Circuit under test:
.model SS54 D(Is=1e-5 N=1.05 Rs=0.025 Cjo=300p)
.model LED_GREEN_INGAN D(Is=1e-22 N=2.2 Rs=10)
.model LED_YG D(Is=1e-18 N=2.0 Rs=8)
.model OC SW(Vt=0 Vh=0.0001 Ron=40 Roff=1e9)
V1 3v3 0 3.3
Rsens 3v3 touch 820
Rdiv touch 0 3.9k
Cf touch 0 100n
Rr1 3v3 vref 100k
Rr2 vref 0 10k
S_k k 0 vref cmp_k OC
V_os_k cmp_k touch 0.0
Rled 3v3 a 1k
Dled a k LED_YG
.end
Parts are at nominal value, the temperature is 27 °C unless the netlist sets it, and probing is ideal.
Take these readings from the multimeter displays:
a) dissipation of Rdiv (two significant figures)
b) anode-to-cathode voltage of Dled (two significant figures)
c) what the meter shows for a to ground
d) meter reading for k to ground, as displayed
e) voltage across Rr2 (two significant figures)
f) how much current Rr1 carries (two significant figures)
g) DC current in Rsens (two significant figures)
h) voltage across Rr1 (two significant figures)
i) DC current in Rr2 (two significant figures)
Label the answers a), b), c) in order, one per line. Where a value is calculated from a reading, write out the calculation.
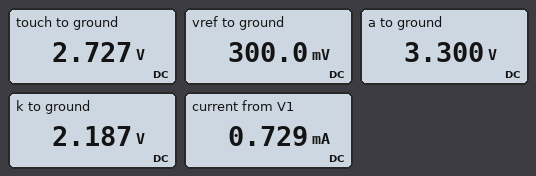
a) (2.727 V)^2 / 3.9 kΩ = 1.9 mW
b) 3.3 V - 2.187 V = 1.1 V
c) 3.300 V
d) 2.187 V
e) 300 mV = 300 mV
f) (3.3 V - 300 mV) / 100 kΩ = 30 µA
g) (3.3 V - 2.727 V) / 820 Ω = 700 µA
h) 3.3 V - 300 mV = 3.0 V
i) (300 mV) / 10 kΩ = 30 µA
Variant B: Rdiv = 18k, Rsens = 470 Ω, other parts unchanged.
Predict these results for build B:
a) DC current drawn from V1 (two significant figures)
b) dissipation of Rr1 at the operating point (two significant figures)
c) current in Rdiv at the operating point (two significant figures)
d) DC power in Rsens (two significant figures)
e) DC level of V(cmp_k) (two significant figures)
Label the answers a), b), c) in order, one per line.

a) 210 µA
b) 90 µW
c) 180 µA
d) 15 µW
e) 3.2 V
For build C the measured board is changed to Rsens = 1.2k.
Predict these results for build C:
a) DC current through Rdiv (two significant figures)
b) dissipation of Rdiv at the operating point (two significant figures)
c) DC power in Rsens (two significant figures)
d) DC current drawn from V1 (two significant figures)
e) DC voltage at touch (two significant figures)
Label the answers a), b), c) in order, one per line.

a) 650 µA
b) 1.6 mW
c) 500 µW
d) 680 µA
e) 2.5 V
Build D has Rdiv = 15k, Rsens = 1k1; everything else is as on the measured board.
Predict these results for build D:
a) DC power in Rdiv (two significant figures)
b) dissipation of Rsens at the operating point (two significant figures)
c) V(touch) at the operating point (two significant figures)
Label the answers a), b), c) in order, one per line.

a) 630 µW
b) 46 µW
c) 3.1 V
